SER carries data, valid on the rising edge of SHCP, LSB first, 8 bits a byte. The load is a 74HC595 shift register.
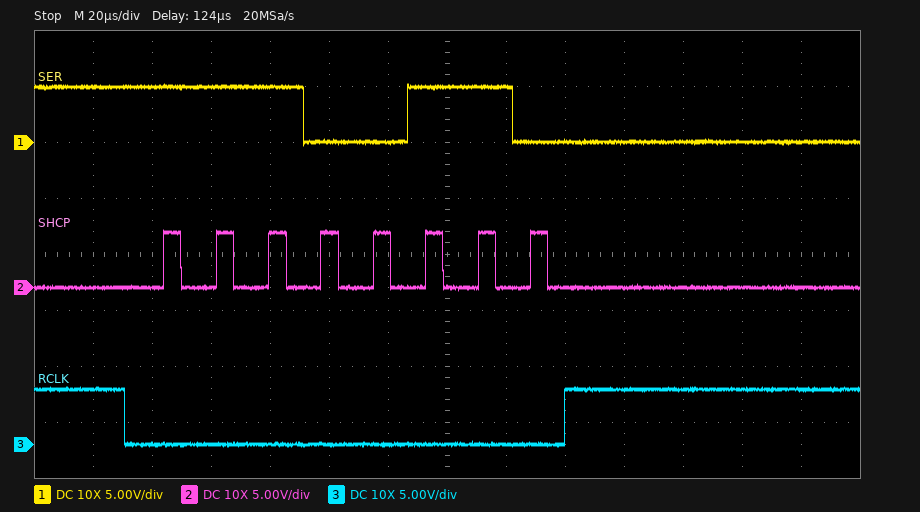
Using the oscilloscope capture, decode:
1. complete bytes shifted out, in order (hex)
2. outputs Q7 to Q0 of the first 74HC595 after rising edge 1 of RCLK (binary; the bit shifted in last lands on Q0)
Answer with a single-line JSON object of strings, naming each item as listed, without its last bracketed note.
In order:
{"complete bytes shifted out, in order": "67", "outputs Q7 to Q0 of the first 74HC595 after rising edge 1 of RCLK": "11100110"}
